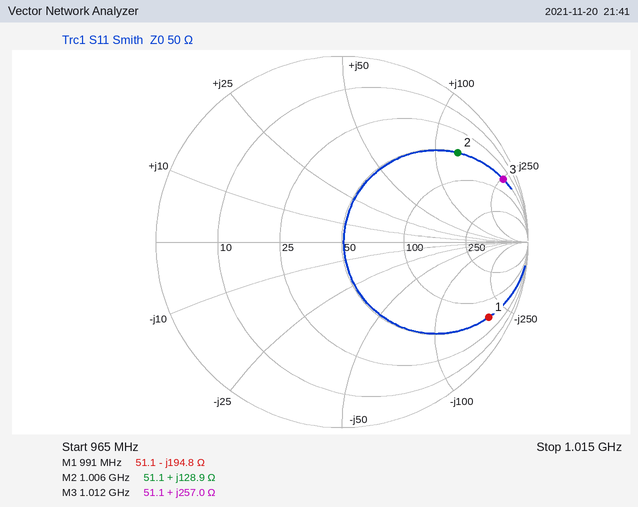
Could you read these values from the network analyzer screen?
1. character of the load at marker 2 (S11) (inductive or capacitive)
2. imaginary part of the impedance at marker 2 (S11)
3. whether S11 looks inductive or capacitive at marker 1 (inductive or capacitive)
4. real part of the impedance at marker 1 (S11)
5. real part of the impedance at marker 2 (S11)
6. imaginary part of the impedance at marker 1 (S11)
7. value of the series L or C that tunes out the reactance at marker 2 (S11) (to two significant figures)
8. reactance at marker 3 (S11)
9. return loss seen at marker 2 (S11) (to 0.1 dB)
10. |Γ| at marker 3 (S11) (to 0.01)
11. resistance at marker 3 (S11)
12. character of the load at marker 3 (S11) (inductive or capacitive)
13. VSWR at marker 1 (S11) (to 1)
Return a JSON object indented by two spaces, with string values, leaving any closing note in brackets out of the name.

{
  "character of the load at marker 2 (S11)": "inductive",
  "imaginary part of the impedance at marker 2": "+128.9 Ω",
  "whether S11 looks inductive or capacitive at marker 1": "capacitive",
  "real part of the impedance at marker 1": "51.1 Ω",
  "real part of the impedance at marker 2": "51.1 Ω",
  "imaginary part of the impedance at marker 1": "-194.8 Ω",
  "value of the series L or C that tunes out the reactance at marker 2 (S11)": "1.2 pF",
  "reactance at marker 3": "+257.0 Ω",
  "return loss seen at marker 2 (S11)": "2.1 dB",
  "|Γ| at marker 3 (S11)": "0.93",
  "resistance at marker 3": "51.1 Ω",
  "character of the load at marker 3 (S11)": "inductive",
  "VSWR at marker 1 (S11)": "17"
}
